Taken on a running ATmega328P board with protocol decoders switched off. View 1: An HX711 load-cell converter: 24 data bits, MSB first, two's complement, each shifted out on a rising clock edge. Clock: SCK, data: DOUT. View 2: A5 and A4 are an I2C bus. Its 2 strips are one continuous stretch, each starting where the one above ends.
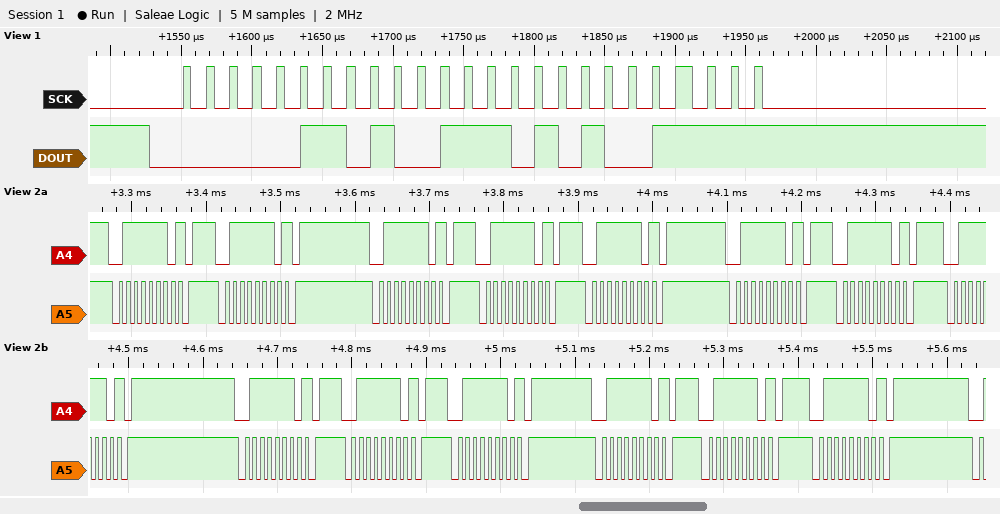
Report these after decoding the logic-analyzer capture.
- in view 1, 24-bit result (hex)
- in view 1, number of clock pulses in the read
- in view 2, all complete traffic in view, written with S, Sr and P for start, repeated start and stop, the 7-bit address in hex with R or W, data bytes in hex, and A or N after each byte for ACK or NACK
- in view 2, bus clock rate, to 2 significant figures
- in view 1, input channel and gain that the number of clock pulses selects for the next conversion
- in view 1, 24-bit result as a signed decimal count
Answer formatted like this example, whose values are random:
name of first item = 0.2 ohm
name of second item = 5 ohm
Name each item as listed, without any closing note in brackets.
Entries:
in view 1, 24-bit result = 0x069D4F
in view 1, number of clock pulses in the read = 25
in view 2, all complete traffic in view, written with S, Sr and P for start, repeated start and stop, the 7-bit address in hex with R or W, data bytes in hex, and A or N after each byte for ACK or NACK = S 3FW N P S 3FW N P S 3FW N P S 3FW N P S 3FW N P S 3FW N P S 3FW N P S 3FW N P S 3FW N P S 3FW N P S 3FW N P S 3FW N P S 3FW N P S 3FW N P
in view 2, bus clock rate, to 2 significant figures = 100 kHz
in view 1, input channel and gain that the number of clock pulses selects for the next conversion = channel A, gain 128
in view 1, 24-bit result as a signed decimal count = 433487
